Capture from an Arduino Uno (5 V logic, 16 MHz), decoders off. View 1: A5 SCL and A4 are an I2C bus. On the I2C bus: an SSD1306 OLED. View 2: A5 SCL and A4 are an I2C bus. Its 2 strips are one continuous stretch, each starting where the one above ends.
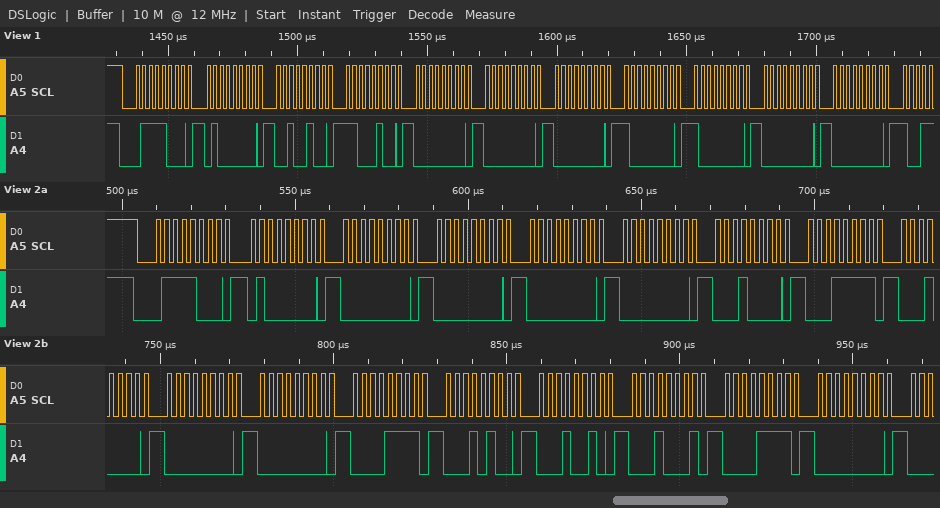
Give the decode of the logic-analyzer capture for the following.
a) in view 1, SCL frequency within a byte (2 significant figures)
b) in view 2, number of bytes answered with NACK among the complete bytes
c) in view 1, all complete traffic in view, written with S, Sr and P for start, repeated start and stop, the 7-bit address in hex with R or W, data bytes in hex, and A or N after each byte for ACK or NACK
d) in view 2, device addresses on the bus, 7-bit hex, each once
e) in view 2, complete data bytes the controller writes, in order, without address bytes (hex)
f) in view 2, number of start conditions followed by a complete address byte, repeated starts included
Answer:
400 kHz
0
S 3CW A 40 A 24 A C4 A 00 A 00 A 00 A 80 A 80 A 00 A 00 A
0x3C
40 00 00 00 00 10 1F 10 00 00 0F 14 12 11 0F 00
1
